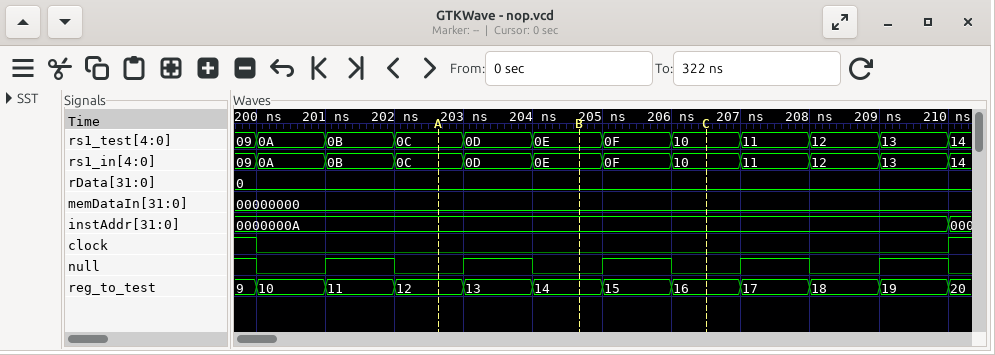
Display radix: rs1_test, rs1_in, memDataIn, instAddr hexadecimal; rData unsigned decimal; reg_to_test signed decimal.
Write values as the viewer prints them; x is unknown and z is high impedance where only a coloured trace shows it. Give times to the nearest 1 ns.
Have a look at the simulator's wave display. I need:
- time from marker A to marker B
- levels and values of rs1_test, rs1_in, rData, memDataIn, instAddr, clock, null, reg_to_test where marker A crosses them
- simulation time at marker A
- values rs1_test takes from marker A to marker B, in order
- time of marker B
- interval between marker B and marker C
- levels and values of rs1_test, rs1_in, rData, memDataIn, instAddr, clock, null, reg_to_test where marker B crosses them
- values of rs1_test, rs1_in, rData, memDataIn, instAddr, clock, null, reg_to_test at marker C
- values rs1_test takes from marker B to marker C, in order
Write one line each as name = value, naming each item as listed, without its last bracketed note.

time from marker A to marker B = 2 ns
levels and values of rs1_test, rs1_in, rData, memDataIn, instAddr, clock, null, reg_to_test where marker A crosses them = rs1_test=0C, rs1_in=0C, rData=0, memDataIn=00000000, instAddr=0000000A, clock=0, null=0, reg_to_test=12
simulation time at marker A = 203 ns
values rs1_test takes from marker A to marker B, in order = 0C, 0D, 0E
time of marker B = 205 ns
interval between marker B and marker C = 2 ns
levels and values of rs1_test, rs1_in, rData, memDataIn, instAddr, clock, null, reg_to_test where marker B crosses them = rs1_test=0E, rs1_in=0E, rData=0, memDataIn=00000000, instAddr=0000000A, clock=0, null=0, reg_to_test=14
values of rs1_test, rs1_in, rData, memDataIn, instAddr, clock, null, reg_to_test at marker C = rs1_test=10, rs1_in=10, rData=0, memDataIn=00000000, instAddr=0000000A, clock=0, null=0, reg_to_test=16
values rs1_test takes from marker B to marker C, in order = 0E, 0F, 10
